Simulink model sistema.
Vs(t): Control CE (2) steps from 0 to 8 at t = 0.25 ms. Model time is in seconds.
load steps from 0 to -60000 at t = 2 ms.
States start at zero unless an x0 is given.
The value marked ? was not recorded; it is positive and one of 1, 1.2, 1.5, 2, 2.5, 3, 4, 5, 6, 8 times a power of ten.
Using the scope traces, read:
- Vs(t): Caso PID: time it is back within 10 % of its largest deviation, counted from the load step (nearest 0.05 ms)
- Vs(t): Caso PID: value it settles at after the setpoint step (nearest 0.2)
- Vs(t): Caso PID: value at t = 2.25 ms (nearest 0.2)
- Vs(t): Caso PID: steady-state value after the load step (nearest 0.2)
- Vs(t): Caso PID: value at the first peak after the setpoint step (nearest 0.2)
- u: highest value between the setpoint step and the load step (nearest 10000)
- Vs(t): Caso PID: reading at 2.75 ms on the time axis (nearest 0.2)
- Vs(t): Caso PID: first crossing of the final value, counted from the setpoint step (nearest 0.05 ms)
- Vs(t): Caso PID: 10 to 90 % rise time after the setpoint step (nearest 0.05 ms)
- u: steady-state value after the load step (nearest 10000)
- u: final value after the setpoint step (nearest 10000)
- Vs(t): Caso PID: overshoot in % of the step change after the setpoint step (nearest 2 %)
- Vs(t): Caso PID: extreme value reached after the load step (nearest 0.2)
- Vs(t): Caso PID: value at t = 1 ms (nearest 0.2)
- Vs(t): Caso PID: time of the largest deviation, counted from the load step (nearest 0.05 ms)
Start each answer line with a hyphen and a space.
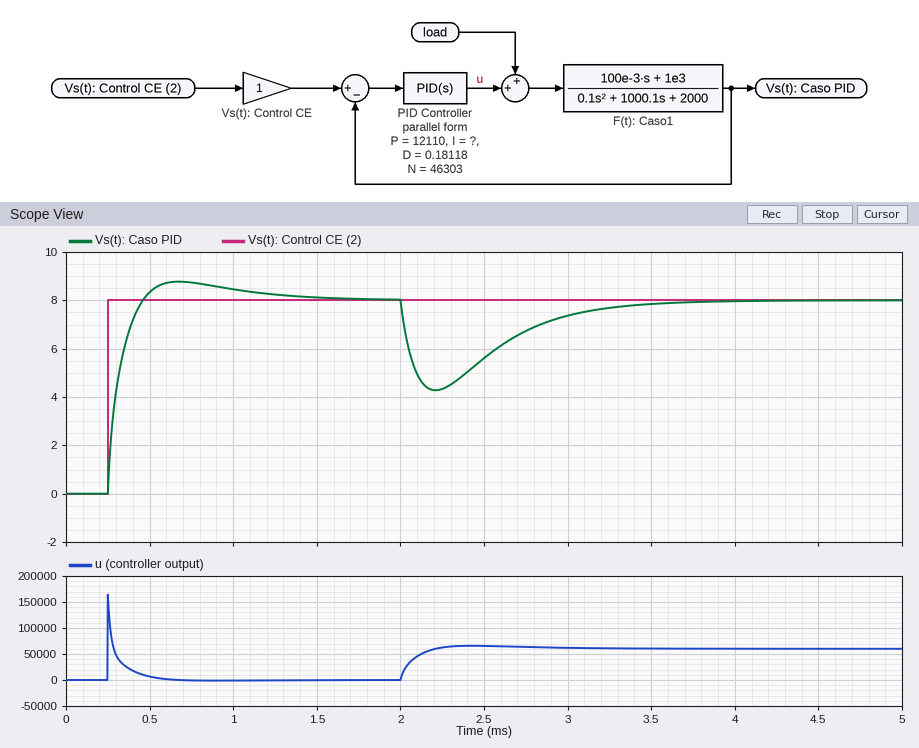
- 1.20 ms
- 8.0
- 4.4
- 8.0
- 8.8
- 160000
- 6.8
- 0.20 ms
- 0.15 ms
- 60000
- 0
- 10 %
- 4.2
- 8.4
- 0.20 ms
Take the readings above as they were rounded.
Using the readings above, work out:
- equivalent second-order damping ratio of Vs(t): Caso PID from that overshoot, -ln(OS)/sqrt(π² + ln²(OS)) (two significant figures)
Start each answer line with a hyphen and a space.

- 0.59
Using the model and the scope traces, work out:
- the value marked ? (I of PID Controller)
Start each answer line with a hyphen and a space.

- 2.5e+07
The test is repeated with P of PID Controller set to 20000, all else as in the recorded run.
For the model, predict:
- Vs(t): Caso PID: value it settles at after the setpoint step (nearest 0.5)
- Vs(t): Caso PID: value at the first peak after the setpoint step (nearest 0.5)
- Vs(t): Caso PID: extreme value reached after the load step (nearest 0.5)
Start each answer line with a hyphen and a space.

- 8.0
- 8.5
- 5.5
